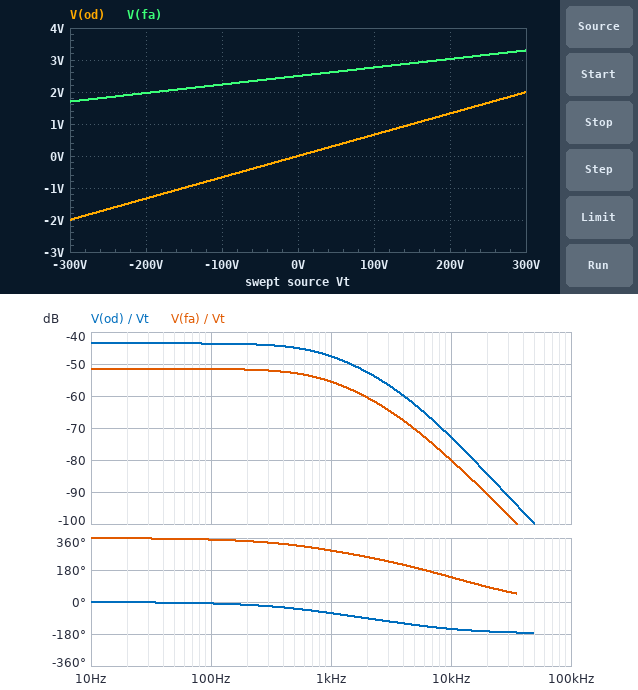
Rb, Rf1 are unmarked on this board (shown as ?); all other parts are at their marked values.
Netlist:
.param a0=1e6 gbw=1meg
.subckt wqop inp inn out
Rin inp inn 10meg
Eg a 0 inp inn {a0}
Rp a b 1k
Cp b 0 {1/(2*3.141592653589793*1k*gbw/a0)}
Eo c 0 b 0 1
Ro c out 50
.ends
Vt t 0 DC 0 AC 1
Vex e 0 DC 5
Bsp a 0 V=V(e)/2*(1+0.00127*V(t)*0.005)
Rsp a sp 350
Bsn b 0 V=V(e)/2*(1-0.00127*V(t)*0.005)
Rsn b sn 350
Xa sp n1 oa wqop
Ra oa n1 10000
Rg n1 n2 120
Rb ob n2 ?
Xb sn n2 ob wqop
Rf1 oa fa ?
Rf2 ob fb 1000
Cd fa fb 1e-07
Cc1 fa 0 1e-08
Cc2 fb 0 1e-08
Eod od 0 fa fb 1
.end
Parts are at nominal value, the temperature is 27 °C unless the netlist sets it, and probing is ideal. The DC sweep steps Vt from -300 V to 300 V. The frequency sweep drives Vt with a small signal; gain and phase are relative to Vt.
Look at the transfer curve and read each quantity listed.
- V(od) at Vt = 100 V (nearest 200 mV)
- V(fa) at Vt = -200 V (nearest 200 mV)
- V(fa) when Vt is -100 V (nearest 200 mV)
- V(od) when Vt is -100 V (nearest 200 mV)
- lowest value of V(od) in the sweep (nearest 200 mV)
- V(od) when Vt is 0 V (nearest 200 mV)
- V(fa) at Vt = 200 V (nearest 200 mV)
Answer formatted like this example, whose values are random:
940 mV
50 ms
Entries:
600 mV
2.0 V
2.2 V
-600 mV
-2.0 V
0 V
3.0 V
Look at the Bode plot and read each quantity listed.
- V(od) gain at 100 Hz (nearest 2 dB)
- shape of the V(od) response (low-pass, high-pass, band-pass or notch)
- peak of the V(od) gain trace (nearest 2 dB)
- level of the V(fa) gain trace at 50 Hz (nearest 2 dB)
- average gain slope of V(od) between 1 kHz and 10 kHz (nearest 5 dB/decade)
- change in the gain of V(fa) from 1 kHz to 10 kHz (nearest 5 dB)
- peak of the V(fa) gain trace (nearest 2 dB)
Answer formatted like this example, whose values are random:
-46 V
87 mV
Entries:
-44 dB
low-pass
-44 dB
-52 dB
-25 dB/decade
-25 dB
-52 dB
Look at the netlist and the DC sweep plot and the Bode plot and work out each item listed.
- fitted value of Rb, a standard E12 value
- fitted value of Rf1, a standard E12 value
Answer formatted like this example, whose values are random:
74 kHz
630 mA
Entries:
15 kΩ
820 Ω
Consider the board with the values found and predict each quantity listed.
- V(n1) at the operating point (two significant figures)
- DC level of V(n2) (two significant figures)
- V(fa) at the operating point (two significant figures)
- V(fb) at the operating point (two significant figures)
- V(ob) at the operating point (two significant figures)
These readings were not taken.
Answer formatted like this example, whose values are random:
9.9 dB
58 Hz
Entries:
2.5 V
2.5 V
2.5 V
2.5 V
2.5 V
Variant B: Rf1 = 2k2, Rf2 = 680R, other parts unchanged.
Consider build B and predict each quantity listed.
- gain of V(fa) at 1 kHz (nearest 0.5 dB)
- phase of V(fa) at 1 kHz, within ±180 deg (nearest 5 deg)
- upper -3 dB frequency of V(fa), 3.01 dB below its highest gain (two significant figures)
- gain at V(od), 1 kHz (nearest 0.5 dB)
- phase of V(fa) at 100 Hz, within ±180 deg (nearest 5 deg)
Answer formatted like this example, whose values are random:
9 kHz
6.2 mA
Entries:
-53.0 dB
-135 deg
2.8 kHz
-50.5 dB
-20 deg
